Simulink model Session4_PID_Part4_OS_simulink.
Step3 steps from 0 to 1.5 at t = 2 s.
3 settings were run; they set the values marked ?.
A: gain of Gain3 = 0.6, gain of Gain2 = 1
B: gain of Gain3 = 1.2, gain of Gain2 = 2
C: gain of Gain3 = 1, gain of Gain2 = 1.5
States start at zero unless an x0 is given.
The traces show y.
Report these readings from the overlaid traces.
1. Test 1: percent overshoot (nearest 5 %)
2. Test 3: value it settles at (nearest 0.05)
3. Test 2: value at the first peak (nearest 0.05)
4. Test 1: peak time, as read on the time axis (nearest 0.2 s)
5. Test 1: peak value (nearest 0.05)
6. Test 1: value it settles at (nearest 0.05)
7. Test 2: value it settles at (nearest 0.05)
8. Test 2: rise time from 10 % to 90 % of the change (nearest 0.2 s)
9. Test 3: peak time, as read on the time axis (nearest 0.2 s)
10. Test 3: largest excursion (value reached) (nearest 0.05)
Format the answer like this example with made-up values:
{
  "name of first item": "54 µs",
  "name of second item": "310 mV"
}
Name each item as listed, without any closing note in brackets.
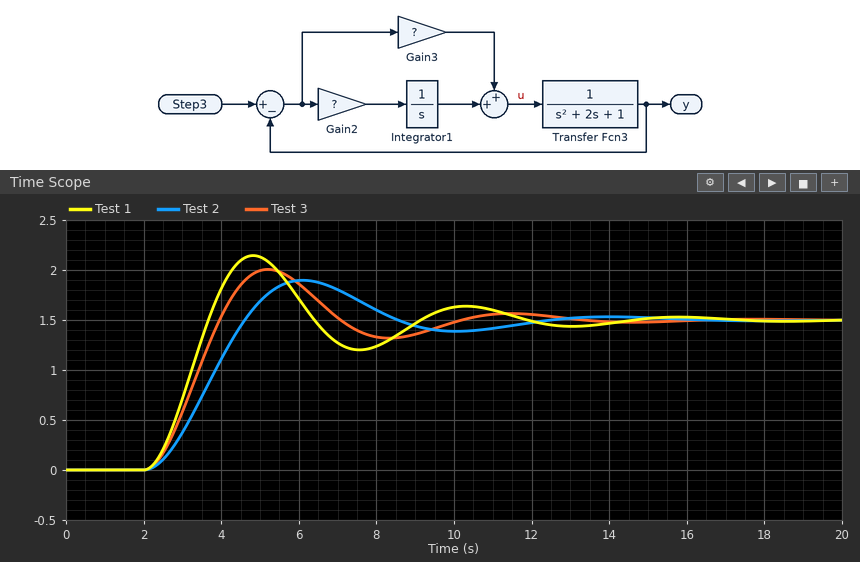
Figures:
{
  "Test 1: percent overshoot": "45 %",
  "Test 3: value it settles at": "1.50",
  "Test 2: value at the first peak": "1.90",
  "Test 1: peak time, as read on the time axis": "4.8 s",
  "Test 1: peak value": "2.15",
  "Test 1: value it settles at": "1.50",
  "Test 2: value it settles at": "1.50",
  "Test 2: rise time from 10 % to 90 % of the change": "1.8 s",
  "Test 3: peak time, as read on the time axis": "5.2 s",
  "Test 3: largest excursion (value reached)": "2.00"
}
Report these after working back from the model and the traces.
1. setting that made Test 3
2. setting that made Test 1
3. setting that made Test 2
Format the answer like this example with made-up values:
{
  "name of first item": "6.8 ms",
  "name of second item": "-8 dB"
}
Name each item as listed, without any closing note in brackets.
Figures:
{
  "setting that made Test 3": "C",
  "setting that made Test 1": "B",
  "setting that made Test 2": "A"
}
